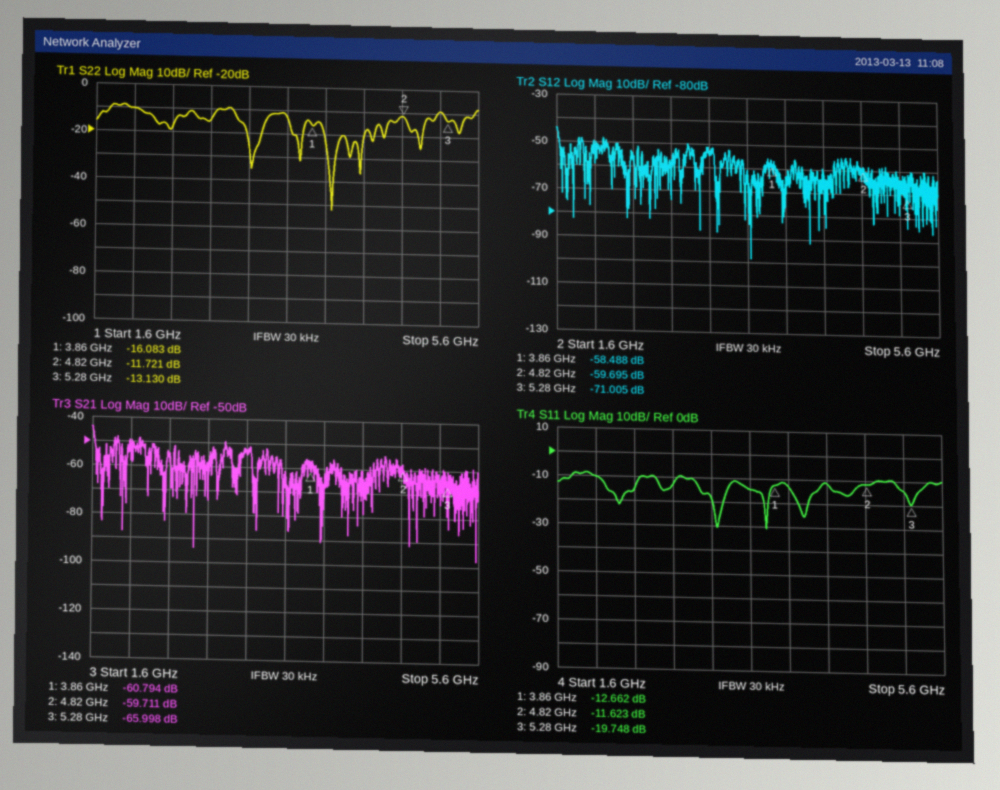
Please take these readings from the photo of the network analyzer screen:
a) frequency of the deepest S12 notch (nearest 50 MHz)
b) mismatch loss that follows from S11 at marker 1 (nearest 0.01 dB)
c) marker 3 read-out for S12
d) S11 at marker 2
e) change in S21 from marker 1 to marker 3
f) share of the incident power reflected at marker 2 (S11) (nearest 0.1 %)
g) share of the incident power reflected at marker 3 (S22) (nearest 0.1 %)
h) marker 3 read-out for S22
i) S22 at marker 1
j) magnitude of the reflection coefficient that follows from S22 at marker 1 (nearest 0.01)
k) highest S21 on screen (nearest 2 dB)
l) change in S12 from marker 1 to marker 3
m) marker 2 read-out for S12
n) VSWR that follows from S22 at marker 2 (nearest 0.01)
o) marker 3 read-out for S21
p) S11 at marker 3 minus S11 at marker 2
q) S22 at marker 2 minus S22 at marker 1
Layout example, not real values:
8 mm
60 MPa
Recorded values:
3.65 GHz
0.24 dB
-71.005 dB
-11.623 dB
-5.204 dB
6.9 %
4.9 %
-13.130 dB
-16.083 dB
0.16
-44 dB
-12.517 dB
-59.695 dB
1.70
-65.998 dB
-8.125 dB
4.362 dB
